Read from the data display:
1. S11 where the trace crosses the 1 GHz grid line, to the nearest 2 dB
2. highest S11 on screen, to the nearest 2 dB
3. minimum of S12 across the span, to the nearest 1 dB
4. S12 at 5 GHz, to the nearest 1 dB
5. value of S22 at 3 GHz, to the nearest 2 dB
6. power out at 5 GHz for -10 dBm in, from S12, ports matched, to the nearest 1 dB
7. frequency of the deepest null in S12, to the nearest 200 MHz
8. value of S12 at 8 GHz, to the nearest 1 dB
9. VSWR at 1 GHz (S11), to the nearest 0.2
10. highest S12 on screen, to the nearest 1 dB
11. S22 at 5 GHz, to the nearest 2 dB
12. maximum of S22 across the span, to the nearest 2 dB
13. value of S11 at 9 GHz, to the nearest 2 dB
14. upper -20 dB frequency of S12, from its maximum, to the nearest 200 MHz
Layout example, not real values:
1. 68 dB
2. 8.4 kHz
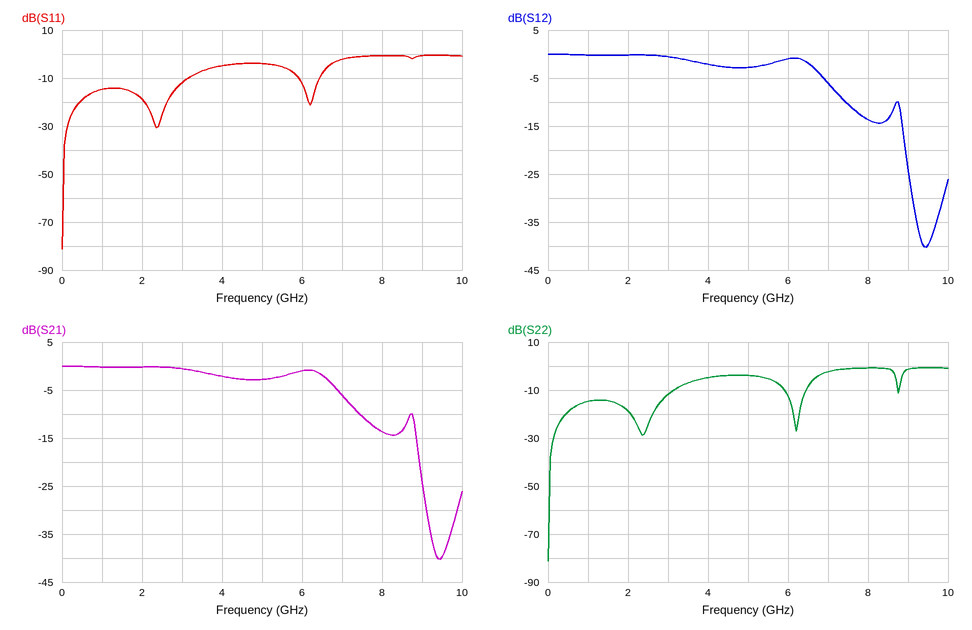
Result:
1. -14 dB
2. 0 dB
3. -40 dB
4. -3 dB
5. -12 dB
6. -13 dBm
7. 9.4 GHz
8. -14 dB
9. 1.4
10. 0 dB
11. -4 dB
12. 0 dB
13. 0 dB
14. 9.0 GHz
